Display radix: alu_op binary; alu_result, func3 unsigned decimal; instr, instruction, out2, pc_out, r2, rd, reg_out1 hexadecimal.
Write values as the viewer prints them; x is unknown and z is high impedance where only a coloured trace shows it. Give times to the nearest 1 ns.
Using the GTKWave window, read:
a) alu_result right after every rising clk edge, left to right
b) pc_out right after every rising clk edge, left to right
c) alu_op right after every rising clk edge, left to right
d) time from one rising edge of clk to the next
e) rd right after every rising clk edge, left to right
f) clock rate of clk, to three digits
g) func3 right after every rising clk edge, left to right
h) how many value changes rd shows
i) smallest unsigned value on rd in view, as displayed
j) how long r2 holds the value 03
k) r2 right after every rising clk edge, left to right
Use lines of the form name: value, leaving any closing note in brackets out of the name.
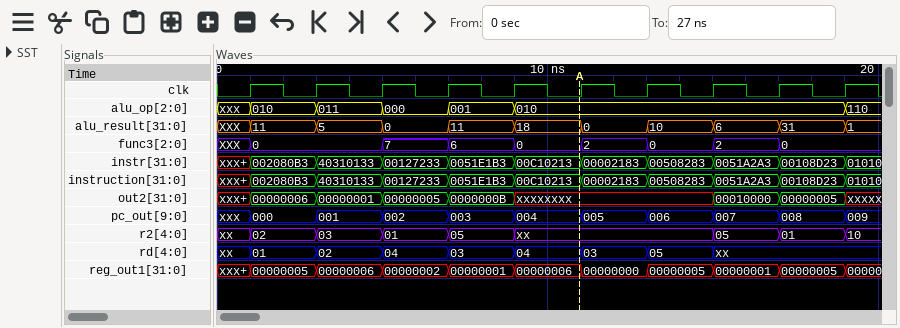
alu_result right after every rising clk edge, left to right: 11, 5, 0, 11, 18, 0, 10, 6, 31, 1
pc_out right after every rising clk edge, left to right: 000, 001, 002, 003, 004, 005, 006, 007, 008, 009
alu_op right after every rising clk edge, left to right: 010, 011, 000, 001, 010, 010, 010, 010, 010, 110
time from one rising edge of clk to the next: 2 ns
rd right after every rising clk edge, left to right: 01, 02, 04, 03, 04, 03, 05, xx, xx, xx
clock rate of clk, to three digits: 500 MHz
func3 right after every rising clk edge, left to right: 0, 0, 7, 6, 0, 2, 0, 2, 0, 0
how many value changes rd shows: 8
smallest unsigned value on rd in view, as displayed: 01
how long r2 holds the value 03: 2 ns
r2 right after every rising clk edge, left to right: 02, 03, 01, 05, xx, xx, xx, 05, 01, 10
